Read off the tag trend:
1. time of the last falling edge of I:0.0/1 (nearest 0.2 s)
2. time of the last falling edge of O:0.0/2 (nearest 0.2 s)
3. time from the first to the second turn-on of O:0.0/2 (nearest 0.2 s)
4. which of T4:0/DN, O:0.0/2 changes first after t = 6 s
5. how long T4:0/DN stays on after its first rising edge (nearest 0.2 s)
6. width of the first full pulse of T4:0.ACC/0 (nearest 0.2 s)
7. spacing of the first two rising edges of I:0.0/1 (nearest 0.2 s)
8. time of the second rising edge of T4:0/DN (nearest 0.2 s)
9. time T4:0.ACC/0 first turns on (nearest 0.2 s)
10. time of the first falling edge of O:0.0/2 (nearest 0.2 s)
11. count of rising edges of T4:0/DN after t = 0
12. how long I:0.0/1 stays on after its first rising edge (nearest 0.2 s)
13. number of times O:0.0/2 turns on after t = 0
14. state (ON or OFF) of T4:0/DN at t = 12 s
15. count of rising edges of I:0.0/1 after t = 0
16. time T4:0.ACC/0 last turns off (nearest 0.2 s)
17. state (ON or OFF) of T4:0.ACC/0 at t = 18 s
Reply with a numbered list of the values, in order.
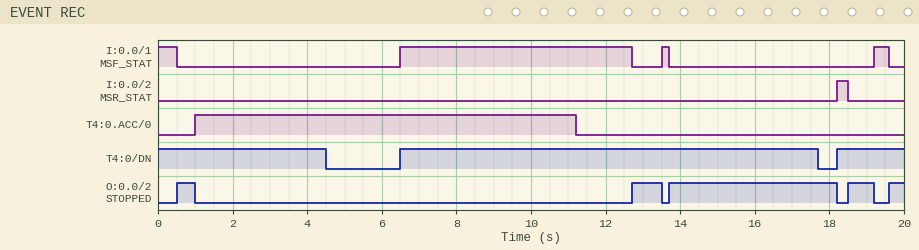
1. 19.6 s
2. 19.2 s
3. 12.2 s
4. T4:0/DN
5. 11.2 s
6. 10.2 s
7. 7.0 s
8. 18.2 s
9. 1.0 s
10. 1.0 s
11. 2
12. 6.2 s
13. 5
14. ON
15. 3
16. 11.2 s
17. OFF
